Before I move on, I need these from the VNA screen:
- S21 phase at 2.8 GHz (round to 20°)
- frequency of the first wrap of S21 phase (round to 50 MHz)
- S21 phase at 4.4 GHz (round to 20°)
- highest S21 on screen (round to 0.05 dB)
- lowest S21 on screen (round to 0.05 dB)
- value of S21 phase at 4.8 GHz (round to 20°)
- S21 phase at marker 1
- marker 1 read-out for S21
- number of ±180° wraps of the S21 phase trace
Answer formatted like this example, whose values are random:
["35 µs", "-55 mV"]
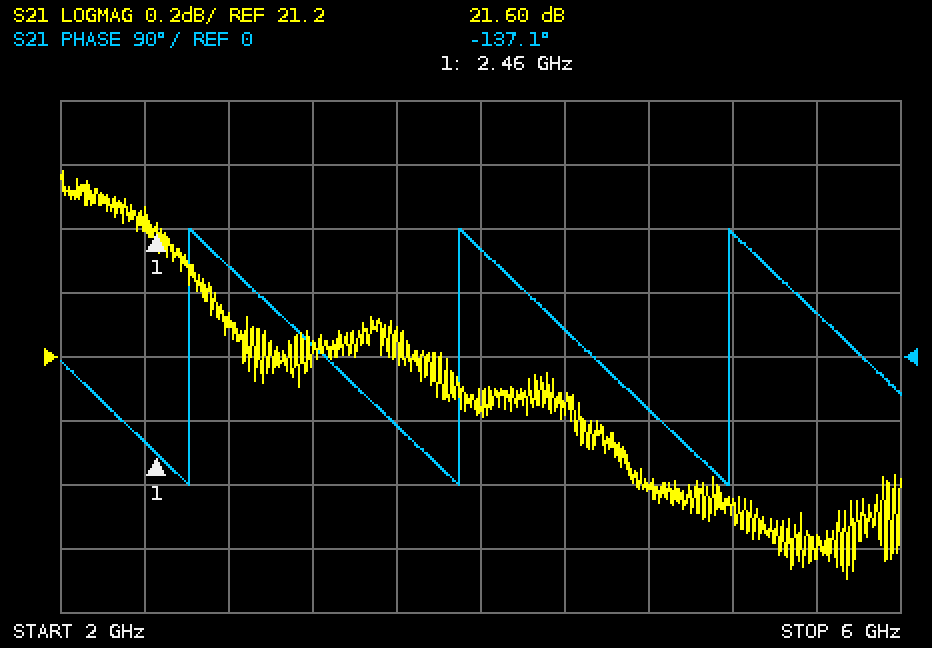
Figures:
["120°", "2.60 GHz", "40°", "21.80 dB", "20.50 dB", "-80°", "-137.1°", "21.60 dB", "3"]
